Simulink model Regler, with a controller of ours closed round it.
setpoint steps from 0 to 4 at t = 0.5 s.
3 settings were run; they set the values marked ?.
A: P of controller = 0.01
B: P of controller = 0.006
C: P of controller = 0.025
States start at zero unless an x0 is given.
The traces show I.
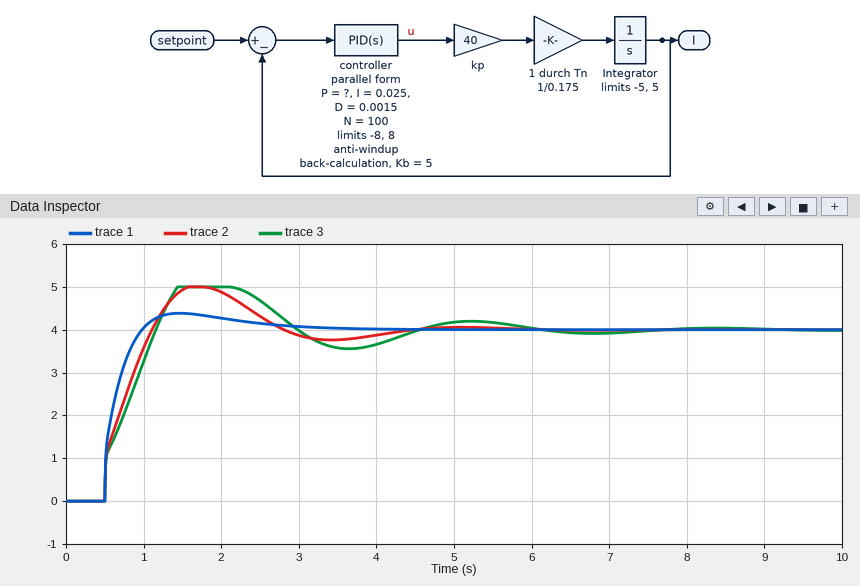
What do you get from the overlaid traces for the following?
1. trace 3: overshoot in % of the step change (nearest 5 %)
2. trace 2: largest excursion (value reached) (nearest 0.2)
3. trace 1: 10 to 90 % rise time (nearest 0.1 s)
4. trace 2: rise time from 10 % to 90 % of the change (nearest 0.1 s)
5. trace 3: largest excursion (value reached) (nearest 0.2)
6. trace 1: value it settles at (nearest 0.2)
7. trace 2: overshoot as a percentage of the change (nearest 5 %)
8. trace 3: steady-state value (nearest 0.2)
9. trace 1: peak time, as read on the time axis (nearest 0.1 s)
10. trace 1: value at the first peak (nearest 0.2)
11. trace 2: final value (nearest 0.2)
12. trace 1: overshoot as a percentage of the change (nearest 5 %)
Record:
25 %
5.0
0.3 s
0.5 s
5.0
4.0
25 %
4.0
1.5 s
4.4
4.0
10 %
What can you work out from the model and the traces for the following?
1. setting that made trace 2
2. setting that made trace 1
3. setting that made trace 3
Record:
A
C
B
